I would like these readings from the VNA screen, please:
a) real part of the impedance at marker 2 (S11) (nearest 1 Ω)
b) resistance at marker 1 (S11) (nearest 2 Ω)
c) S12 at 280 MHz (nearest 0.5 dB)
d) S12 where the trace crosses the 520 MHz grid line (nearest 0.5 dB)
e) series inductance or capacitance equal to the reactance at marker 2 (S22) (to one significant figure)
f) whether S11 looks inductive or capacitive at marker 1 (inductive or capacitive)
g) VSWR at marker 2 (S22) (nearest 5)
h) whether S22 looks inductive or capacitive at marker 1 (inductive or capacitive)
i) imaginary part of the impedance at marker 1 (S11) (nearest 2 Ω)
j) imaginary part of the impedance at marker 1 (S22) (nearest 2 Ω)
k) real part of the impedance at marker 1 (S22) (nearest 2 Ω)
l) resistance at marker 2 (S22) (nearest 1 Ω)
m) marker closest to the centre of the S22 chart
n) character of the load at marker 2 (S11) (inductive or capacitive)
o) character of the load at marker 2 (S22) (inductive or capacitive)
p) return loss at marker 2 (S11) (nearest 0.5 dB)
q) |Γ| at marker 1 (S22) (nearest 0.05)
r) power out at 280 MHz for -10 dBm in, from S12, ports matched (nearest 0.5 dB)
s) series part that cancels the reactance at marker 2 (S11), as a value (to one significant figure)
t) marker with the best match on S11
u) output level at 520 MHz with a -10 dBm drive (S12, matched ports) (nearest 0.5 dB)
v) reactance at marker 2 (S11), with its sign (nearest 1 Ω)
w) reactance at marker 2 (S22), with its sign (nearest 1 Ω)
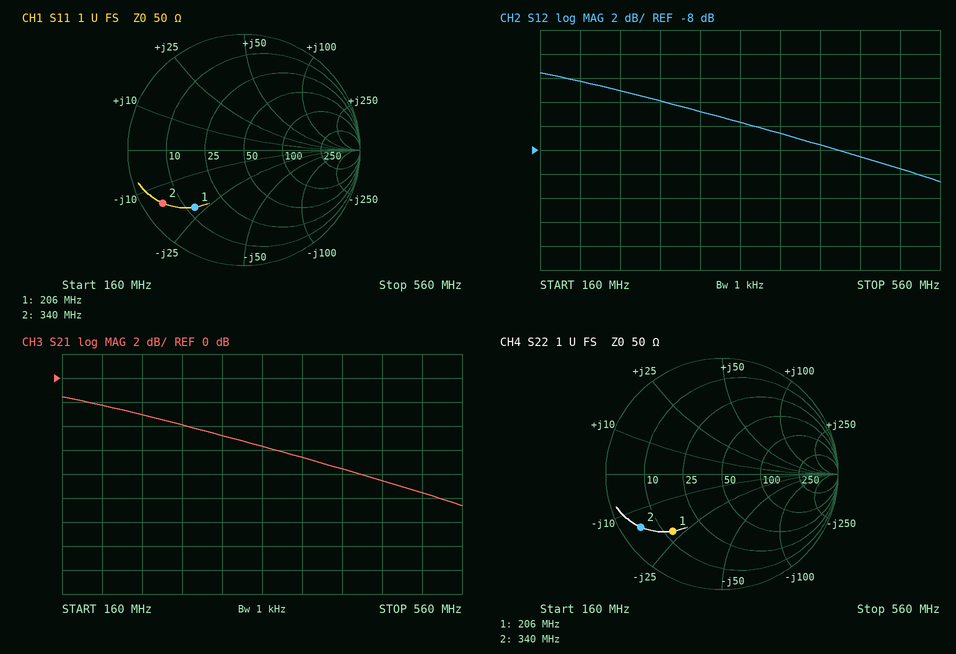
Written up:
5 Ω
12 Ω
-4.0 dB
-9.5 dB
30 pF
capacitive
10
capacitive
-22 Ω
-22 Ω
12 Ω
5 Ω
marker 1
capacitive
capacitive
1.5 dB
0.65
-14.0 dBm
7 nH
marker 1
-19.5 dBm
-15 Ω
-15 Ω
